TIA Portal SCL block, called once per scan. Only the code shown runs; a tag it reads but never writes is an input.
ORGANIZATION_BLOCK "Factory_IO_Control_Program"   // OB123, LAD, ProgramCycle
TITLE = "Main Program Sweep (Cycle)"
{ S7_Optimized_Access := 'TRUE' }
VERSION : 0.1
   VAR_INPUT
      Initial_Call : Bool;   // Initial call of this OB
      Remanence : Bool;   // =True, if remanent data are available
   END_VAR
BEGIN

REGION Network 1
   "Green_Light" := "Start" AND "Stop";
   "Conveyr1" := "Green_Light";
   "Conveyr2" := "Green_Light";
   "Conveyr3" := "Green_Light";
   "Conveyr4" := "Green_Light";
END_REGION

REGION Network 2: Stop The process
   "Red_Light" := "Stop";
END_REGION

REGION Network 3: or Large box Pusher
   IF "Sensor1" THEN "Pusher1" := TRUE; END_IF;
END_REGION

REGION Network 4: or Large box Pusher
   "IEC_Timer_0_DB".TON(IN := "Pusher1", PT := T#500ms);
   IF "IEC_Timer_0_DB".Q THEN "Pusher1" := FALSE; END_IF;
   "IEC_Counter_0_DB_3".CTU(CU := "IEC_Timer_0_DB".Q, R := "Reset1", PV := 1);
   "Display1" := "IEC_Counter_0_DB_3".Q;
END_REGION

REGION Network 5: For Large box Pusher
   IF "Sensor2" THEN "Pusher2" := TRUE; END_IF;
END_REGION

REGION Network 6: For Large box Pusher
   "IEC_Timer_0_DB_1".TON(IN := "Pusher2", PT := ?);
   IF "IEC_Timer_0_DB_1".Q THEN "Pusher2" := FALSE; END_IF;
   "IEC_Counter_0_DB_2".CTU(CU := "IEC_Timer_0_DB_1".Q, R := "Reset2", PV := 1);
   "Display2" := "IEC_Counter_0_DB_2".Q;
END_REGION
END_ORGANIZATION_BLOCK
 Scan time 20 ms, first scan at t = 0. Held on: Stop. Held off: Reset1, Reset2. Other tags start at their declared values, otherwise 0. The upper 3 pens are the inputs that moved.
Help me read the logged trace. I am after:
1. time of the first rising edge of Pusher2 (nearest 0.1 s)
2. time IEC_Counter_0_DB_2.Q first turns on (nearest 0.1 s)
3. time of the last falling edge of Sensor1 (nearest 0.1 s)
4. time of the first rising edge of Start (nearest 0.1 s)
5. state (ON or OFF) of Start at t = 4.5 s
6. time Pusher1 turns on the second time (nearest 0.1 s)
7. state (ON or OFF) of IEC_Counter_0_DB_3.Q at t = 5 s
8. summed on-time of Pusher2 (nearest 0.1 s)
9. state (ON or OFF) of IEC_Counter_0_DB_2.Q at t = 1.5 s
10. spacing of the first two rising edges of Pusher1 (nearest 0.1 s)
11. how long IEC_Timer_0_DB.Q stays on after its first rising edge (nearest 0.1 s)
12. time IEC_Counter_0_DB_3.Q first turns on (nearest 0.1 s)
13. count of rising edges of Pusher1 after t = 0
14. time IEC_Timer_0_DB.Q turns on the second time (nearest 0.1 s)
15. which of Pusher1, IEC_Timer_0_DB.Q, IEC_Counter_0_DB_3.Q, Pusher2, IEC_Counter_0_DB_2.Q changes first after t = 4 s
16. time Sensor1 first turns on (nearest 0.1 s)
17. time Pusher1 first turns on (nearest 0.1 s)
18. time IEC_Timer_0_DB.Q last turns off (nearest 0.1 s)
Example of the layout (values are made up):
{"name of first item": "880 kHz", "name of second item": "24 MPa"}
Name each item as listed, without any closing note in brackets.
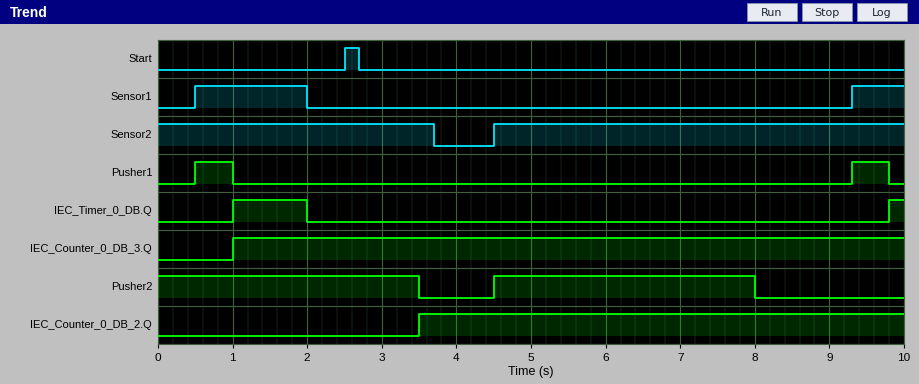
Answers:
{"time of the first rising edge of Pusher2": "4.5 s", "time IEC_Counter_0_DB_2.Q first turns on": "3.5 s", "time of the last falling edge of Sensor1": "2.0 s", "time of the first rising edge of Start": "2.5 s", "state (ON or OFF) of Start at t = 4.5 s": "OFF", "time Pusher1 turns on the second time": "9.3 s", "state (ON or OFF) of IEC_Counter_0_DB_3.Q at t = 5 s": "ON", "summed on-time of Pusher2": "7.0 s", "state (ON or OFF) of IEC_Counter_0_DB_2.Q at t = 1.5 s": "OFF", "spacing of the first two rising edges of Pusher1": "8.8 s", "how long IEC_Timer_0_DB.Q stays on after its first rising edge": "1.0 s", "time IEC_Counter_0_DB_3.Q first turns on": "1.0 s", "count of rising edges of Pusher1 after t = 0": "2", "time IEC_Timer_0_DB.Q turns on the second time": "9.8 s", "which of Pusher1, IEC_Timer_0_DB.Q, IEC_Counter_0_DB_3.Q, Pusher2, IEC_Counter_0_DB_2.Q changes first after t = 4 s": "Pusher2", "time Sensor1 first turns on": "0.5 s", "time Pusher1 first turns on": "0.5 s", "time IEC_Timer_0_DB.Q last turns off": "2.0 s"}
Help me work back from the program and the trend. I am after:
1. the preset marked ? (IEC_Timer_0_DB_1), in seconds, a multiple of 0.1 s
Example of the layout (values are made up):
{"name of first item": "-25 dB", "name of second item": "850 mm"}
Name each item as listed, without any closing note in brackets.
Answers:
{"the preset marked ? (IEC_Timer_0_DB_1), in seconds, a multiple of 0.1 s": "3.5 s"}
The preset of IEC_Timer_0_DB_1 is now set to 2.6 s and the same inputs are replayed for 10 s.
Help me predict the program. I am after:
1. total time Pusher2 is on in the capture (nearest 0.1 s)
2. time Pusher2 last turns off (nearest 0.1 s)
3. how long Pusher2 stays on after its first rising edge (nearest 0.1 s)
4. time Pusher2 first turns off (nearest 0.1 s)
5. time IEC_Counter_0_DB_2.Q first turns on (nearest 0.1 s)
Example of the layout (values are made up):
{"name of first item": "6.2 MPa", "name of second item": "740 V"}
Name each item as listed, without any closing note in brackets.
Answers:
{"total time Pusher2 is on in the capture": "5.2 s", "time Pusher2 last turns off": "7.1 s", "how long Pusher2 stays on after its first rising edge": "2.6 s", "time Pusher2 first turns off": "2.6 s", "time IEC_Counter_0_DB_2.Q first turns on": "2.6 s"}
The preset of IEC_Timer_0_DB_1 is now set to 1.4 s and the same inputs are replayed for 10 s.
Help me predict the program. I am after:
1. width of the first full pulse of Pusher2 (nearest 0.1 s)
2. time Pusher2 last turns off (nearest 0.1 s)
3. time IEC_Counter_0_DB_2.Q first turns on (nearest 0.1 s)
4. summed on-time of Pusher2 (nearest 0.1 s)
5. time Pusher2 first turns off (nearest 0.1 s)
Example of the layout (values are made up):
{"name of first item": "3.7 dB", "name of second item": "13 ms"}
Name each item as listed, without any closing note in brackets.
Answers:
{"width of the first full pulse of Pusher2": "1.4 s", "time Pusher2 last turns off": "5.9 s", "time IEC_Counter_0_DB_2.Q first turns on": "1.4 s", "summed on-time of Pusher2": "2.8 s", "time Pusher2 first turns off": "1.4 s"}
